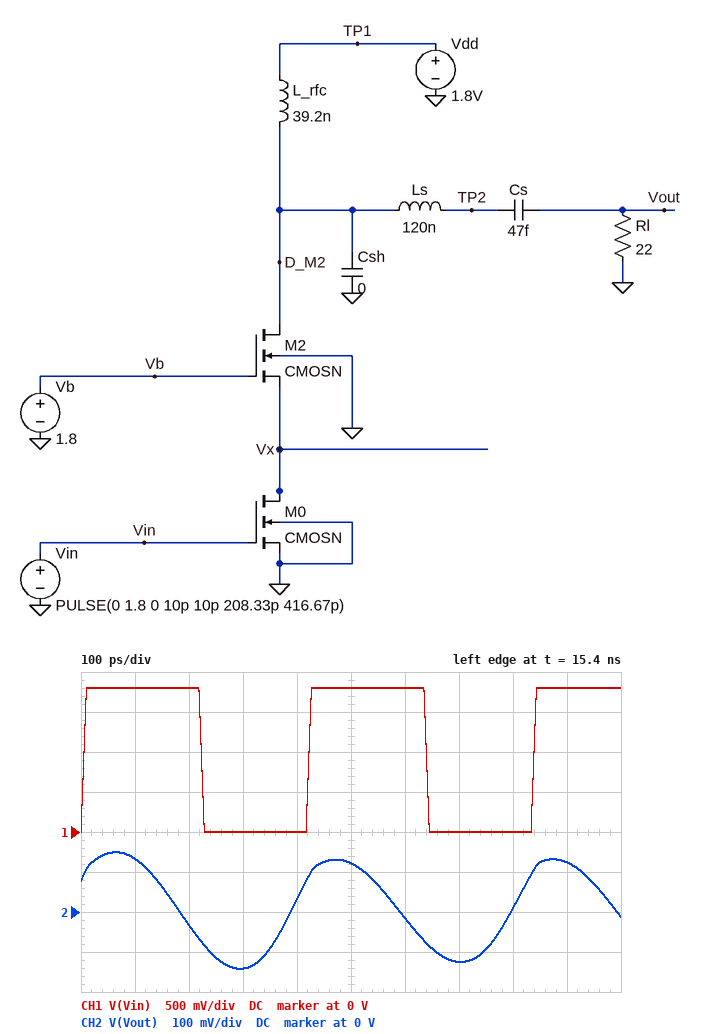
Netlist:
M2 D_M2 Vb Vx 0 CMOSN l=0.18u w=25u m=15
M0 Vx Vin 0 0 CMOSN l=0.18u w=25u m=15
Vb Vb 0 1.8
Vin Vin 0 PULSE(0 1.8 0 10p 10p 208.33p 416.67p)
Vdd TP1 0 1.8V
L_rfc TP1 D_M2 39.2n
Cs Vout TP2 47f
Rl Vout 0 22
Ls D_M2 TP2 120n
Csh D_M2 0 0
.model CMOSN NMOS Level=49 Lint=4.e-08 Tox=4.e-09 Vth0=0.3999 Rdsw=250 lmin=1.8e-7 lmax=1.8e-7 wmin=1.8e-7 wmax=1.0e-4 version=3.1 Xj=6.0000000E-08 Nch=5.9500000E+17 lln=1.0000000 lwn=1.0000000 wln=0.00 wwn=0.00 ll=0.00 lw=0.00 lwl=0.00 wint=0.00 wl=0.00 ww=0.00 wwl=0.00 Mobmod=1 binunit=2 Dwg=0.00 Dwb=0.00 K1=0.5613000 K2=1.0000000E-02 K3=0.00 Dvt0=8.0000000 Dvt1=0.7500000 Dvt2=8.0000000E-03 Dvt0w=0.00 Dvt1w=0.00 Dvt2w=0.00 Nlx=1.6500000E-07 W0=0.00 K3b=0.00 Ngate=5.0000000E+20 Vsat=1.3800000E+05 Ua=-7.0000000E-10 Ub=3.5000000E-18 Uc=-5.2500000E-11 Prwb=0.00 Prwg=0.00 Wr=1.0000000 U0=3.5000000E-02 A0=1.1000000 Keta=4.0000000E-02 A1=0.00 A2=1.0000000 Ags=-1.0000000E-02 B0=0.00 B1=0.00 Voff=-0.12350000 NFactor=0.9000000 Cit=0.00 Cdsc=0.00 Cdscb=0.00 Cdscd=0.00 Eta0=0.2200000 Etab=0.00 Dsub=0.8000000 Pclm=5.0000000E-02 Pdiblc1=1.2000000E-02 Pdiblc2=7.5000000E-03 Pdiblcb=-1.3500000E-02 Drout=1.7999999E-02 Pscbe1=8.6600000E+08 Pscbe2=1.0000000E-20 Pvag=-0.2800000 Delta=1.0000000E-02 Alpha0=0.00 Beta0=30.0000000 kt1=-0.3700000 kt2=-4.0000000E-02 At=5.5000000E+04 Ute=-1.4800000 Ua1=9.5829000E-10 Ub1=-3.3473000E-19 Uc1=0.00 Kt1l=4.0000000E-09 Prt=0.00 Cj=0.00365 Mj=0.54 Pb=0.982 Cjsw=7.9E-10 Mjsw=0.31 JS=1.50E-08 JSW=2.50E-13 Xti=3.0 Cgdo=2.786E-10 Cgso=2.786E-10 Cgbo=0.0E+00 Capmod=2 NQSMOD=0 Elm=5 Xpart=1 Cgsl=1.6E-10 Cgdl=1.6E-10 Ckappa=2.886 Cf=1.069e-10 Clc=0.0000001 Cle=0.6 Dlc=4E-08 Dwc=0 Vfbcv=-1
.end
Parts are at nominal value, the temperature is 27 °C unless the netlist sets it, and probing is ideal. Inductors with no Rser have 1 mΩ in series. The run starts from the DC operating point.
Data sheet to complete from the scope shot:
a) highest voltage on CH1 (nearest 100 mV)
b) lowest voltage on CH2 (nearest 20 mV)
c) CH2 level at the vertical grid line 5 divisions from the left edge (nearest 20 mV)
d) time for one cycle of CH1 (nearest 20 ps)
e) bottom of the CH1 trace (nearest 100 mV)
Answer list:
1.8 V
-140 mV
120 mV
420 ps
0 V
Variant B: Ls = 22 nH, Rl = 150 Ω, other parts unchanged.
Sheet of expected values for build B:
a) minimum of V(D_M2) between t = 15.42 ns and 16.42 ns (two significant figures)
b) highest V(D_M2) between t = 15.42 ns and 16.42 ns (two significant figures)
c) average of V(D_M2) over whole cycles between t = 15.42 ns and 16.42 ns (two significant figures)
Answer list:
-130 mV
7.6 V
1.8 V
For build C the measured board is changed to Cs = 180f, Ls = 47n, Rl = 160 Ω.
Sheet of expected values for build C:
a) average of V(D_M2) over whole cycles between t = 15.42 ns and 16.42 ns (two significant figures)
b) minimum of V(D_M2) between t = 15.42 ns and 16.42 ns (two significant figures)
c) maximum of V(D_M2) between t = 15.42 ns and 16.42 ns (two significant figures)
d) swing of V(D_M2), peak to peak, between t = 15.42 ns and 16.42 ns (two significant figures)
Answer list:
1.8 V
-120 mV
7.3 V
7.4 V
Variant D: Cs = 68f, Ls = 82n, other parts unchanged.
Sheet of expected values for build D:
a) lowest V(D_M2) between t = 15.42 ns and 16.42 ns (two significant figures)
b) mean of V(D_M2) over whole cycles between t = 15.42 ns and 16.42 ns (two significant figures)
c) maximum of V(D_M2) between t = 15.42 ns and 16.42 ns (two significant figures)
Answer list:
-130 mV
1.8 V
7.1 V
